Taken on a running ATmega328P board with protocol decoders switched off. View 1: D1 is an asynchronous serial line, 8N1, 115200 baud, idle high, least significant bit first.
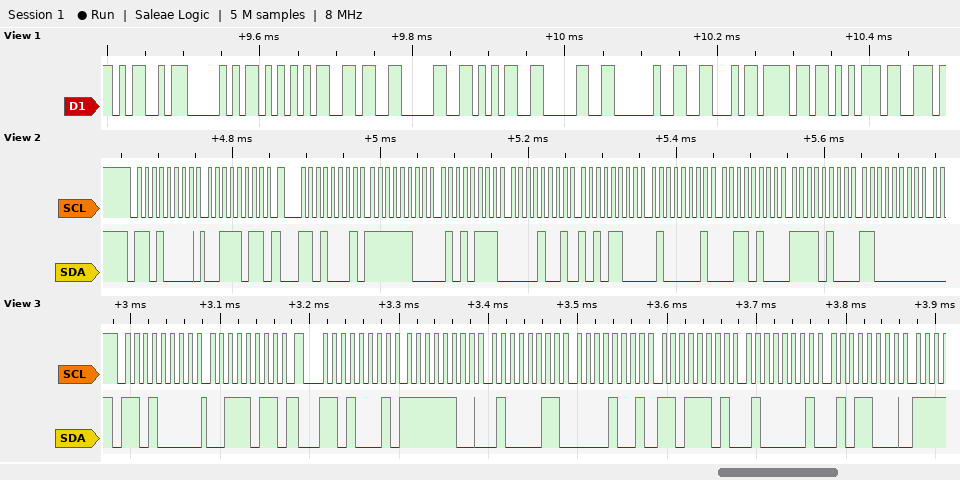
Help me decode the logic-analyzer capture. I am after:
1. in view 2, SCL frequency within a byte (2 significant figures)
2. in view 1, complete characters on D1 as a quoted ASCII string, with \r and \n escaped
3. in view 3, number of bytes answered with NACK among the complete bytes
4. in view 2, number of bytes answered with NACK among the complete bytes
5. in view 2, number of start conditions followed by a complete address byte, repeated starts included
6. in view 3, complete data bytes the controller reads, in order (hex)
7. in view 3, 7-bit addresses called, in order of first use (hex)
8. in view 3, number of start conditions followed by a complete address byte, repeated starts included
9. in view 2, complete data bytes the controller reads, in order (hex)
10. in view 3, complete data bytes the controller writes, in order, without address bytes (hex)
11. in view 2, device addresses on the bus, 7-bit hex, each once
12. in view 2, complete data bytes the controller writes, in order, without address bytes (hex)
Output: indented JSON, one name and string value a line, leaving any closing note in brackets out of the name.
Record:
{
  "in view 2, SCL frequency within a byte": "100 kHz",
  "in view 1, complete characters on D1 as a quoted ASCII string, with \\r and \\n escaped": "\"MPU6050 Fou\"",
  "in view 3, number of bytes answered with NACK among the complete bytes": "0",
  "in view 2, number of bytes answered with NACK among the complete bytes": "0",
  "in view 2, number of start conditions followed by a complete address byte, repeated starts included": "2",
  "in view 3, complete data bytes the controller reads, in order": "FC 43 09 DD 41 58",
  "in view 3, 7-bit addresses called, in order of first use": "0x68",
  "in view 3, number of start conditions followed by a complete address byte, repeated starts included": "2",
  "in view 2, complete data bytes the controller reads, in order": "FC 57 09 AC 41 34 F4 C0",
  "in view 3, complete data bytes the controller writes, in order, without address bytes": "3B",
  "in view 2, device addresses on the bus, 7-bit hex, each once": "0x68",
  "in view 2, complete data bytes the controller writes, in order, without address bytes": "3B"
}
